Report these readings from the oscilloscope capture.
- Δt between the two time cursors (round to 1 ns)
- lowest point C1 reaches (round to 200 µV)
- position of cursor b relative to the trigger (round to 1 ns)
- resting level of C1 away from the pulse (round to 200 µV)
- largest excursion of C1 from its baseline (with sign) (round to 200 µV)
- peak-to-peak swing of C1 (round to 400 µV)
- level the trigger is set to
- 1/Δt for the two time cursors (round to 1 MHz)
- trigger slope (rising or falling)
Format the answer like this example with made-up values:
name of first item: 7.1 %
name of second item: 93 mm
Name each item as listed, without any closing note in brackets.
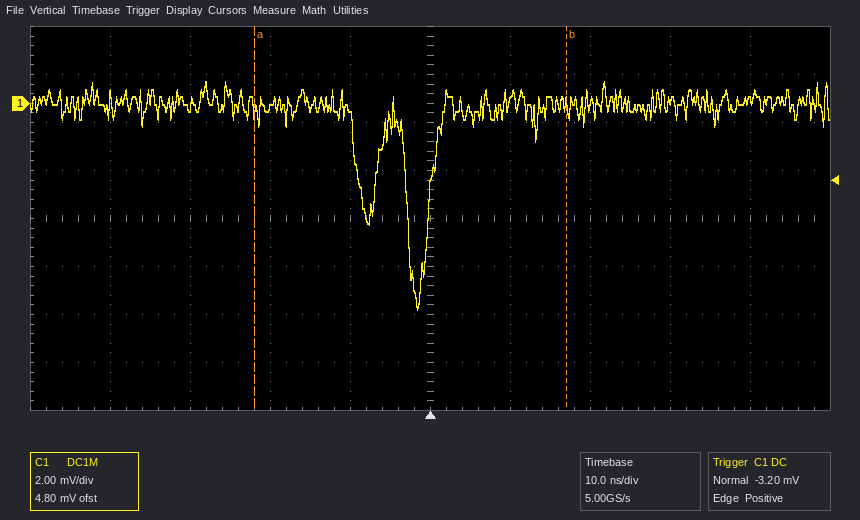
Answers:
Δt between the two time cursors: 39 ns
lowest point C1 reaches: -8.6 mV
position of cursor b relative to the trigger: +17 ns
resting level of C1 away from the pulse: 0.0 mV
largest excursion of C1 from its baseline (with sign): -8.6 mV
peak-to-peak swing of C1: 9.6 mV
level the trigger is set to: -3.20 mV
1/Δt for the two time cursors: 26 MHz
trigger slope: rising
